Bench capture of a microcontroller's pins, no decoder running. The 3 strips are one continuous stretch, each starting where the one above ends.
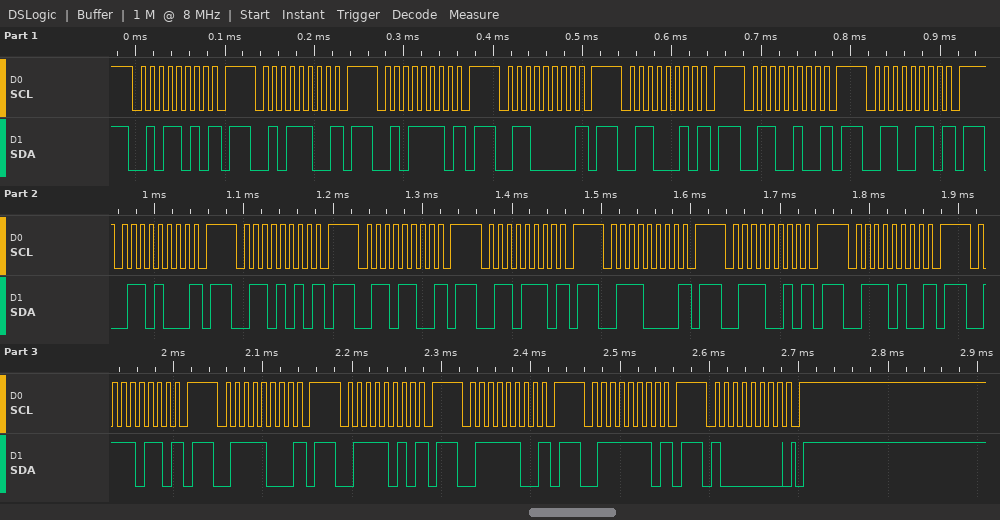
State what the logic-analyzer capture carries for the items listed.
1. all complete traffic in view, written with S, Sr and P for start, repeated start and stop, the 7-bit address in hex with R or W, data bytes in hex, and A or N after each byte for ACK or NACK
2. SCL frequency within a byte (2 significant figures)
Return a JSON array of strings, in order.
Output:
["S 2DW N P S 2EW N P S 2FW N P S 30W N P S 31W N P S 32W N P S 33W N P S 34W N P S 35W N P S 36W N P S 37W N P S 38W N P S 39W N P S 3AW N P S 3BW N P S 3CW N P S 3DW N P S 3EW N P S 3FW N P S 40W A P", "100 kHz"]
